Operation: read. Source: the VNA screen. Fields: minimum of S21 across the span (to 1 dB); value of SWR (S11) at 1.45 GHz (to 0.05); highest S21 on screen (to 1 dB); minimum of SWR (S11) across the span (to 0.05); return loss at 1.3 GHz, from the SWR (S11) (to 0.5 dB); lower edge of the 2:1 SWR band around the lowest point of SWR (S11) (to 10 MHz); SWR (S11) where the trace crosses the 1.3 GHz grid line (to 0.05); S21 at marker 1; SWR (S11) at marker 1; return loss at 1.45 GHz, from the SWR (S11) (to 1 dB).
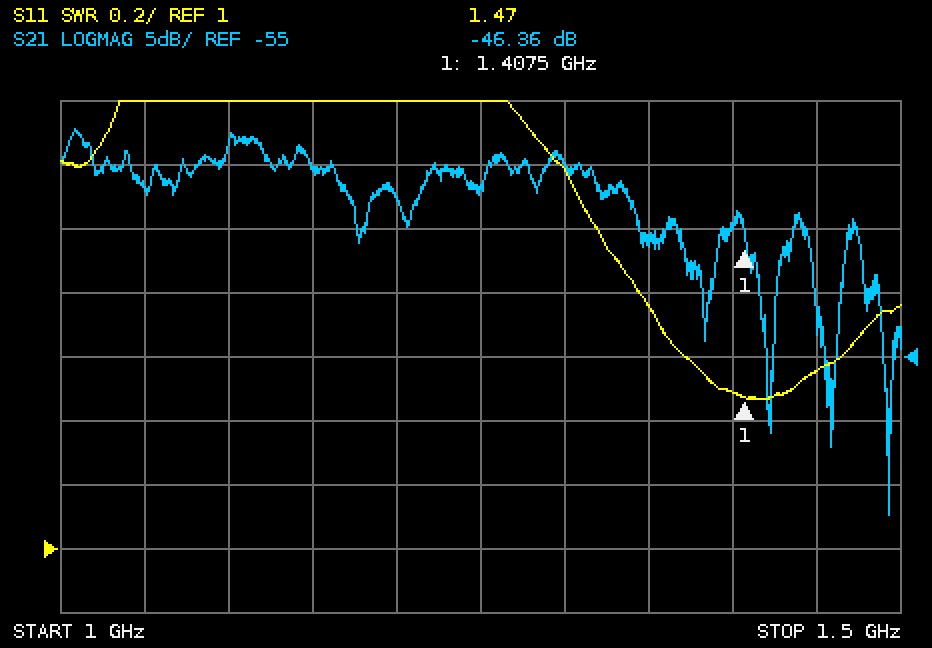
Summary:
-67 dB
1.55
-37 dB
1.45
8.5 dB
1.32 GHz
2.20
-46.36 dB
1.47
13 dB
